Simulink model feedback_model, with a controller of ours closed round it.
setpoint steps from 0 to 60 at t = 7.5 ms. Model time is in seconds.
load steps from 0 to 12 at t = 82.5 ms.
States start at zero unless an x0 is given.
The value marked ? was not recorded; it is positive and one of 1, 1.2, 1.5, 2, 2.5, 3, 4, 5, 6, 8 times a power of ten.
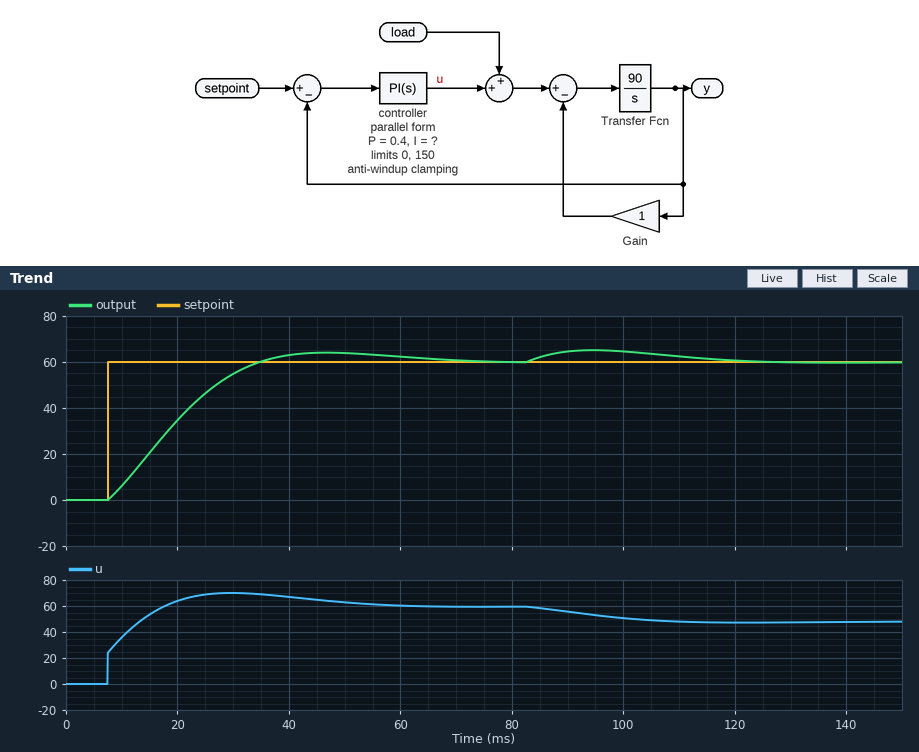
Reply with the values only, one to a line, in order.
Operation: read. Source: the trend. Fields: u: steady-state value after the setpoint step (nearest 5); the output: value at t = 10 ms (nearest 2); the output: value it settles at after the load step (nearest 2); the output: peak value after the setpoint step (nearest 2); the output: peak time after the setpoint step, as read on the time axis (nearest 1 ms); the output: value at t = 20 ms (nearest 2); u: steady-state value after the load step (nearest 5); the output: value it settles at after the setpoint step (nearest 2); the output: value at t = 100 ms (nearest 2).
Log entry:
60
6
60
64
47 ms
34
50
60
64
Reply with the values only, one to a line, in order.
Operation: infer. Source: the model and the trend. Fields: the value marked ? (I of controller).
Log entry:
100
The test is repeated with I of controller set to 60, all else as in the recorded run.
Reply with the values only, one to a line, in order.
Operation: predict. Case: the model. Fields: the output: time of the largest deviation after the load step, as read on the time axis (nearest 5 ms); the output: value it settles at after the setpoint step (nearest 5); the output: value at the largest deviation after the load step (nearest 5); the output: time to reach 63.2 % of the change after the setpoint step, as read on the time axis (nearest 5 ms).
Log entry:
95 ms
60
65
25 ms
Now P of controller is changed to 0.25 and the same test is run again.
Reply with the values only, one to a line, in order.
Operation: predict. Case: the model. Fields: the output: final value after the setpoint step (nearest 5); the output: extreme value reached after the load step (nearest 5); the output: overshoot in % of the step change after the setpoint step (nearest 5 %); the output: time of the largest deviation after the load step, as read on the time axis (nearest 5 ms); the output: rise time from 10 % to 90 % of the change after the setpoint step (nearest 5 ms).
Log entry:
60
65
10 %
95 ms
20 ms
